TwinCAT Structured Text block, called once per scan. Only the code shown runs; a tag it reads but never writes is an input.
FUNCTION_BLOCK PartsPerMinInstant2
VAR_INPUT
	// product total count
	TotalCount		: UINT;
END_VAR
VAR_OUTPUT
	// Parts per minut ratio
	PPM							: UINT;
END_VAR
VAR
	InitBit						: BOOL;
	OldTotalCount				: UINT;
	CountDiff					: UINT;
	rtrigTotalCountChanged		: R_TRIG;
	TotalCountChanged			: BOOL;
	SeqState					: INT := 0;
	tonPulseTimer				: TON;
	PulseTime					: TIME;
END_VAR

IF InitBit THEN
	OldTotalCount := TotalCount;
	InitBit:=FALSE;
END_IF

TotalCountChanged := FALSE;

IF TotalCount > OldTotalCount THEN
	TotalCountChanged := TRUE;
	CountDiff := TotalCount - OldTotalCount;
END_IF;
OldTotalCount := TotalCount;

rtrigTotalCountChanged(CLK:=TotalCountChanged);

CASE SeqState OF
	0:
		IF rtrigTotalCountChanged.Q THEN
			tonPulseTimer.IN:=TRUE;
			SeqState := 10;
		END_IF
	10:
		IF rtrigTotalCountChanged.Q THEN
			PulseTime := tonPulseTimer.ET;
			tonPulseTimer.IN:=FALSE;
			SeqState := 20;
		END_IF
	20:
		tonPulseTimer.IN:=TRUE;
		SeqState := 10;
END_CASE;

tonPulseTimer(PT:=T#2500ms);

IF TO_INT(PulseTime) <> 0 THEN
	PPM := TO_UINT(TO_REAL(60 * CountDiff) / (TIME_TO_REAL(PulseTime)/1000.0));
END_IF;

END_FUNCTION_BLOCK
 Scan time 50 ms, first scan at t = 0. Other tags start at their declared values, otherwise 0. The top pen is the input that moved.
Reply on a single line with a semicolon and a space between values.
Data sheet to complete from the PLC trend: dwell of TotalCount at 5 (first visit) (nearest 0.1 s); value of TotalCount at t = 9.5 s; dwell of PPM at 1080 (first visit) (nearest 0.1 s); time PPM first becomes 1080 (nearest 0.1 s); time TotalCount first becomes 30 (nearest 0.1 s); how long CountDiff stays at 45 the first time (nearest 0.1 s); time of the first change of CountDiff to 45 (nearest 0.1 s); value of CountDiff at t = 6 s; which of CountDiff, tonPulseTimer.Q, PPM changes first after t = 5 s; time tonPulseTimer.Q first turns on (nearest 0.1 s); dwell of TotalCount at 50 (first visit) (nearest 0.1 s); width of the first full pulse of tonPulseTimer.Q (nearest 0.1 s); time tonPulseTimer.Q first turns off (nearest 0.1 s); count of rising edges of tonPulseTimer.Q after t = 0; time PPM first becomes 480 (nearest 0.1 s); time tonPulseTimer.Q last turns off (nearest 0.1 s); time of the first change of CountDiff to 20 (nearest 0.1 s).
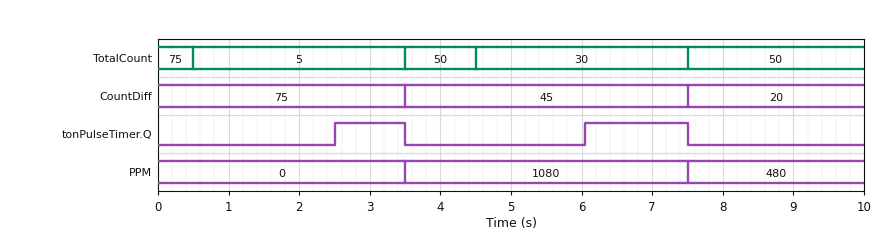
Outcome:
3.0 s; 50; 4.0 s; 3.5 s; 4.5 s; 4.0 s; 3.5 s; 45; tonPulseTimer.Q; 2.5 s; 1.0 s; 1.0 s; 3.5 s; 2; 7.5 s; 7.5 s; 7.5 s
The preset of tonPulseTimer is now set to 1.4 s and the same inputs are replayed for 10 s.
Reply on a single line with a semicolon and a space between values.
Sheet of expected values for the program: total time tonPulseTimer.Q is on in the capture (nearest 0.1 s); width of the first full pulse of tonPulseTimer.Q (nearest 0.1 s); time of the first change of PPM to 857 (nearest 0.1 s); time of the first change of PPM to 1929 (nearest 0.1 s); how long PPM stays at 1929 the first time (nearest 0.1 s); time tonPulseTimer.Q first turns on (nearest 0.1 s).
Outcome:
5.7 s; 2.1 s; 7.5 s; 3.5 s; 4.0 s; 1.4 s
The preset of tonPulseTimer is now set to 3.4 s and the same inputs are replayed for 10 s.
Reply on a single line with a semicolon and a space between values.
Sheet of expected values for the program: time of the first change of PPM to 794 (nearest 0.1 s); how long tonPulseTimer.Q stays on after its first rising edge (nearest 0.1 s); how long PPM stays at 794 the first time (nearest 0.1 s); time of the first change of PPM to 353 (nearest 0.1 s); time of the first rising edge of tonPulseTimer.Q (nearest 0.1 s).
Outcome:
3.5 s; 0.1 s; 4.0 s; 7.5 s; 3.4 s
